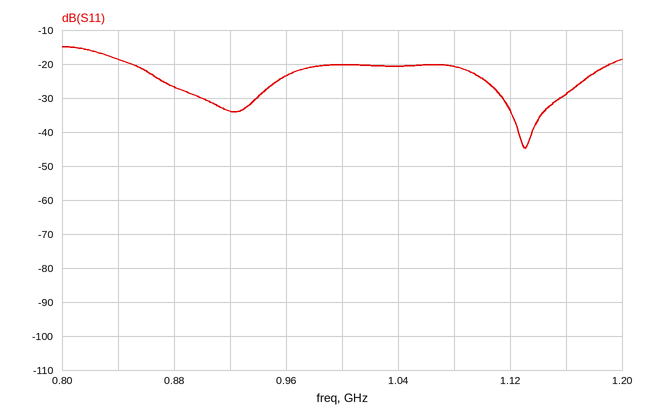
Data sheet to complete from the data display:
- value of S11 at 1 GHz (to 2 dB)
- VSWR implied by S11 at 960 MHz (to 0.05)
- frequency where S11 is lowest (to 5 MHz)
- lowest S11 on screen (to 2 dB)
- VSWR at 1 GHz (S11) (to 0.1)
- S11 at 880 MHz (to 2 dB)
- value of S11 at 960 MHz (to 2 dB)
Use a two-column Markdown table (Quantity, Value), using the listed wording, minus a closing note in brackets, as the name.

| Quantity | Value |
|---|---|
| value of S11 at 1 GHz | -20 dB |
| VSWR implied by S11 at 960 MHz | 1.15 |
| frequency where S11 is lowest | 1.130 GHz |
| lowest S11 on screen | -44 dB |
| VSWR at 1 GHz (S11) | 1.2 |
| S11 at 880 MHz | -26 dB |
| value of S11 at 960 MHz | -24 dB |
